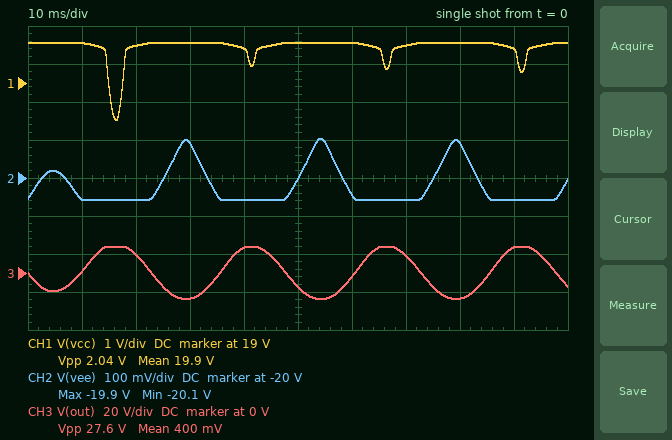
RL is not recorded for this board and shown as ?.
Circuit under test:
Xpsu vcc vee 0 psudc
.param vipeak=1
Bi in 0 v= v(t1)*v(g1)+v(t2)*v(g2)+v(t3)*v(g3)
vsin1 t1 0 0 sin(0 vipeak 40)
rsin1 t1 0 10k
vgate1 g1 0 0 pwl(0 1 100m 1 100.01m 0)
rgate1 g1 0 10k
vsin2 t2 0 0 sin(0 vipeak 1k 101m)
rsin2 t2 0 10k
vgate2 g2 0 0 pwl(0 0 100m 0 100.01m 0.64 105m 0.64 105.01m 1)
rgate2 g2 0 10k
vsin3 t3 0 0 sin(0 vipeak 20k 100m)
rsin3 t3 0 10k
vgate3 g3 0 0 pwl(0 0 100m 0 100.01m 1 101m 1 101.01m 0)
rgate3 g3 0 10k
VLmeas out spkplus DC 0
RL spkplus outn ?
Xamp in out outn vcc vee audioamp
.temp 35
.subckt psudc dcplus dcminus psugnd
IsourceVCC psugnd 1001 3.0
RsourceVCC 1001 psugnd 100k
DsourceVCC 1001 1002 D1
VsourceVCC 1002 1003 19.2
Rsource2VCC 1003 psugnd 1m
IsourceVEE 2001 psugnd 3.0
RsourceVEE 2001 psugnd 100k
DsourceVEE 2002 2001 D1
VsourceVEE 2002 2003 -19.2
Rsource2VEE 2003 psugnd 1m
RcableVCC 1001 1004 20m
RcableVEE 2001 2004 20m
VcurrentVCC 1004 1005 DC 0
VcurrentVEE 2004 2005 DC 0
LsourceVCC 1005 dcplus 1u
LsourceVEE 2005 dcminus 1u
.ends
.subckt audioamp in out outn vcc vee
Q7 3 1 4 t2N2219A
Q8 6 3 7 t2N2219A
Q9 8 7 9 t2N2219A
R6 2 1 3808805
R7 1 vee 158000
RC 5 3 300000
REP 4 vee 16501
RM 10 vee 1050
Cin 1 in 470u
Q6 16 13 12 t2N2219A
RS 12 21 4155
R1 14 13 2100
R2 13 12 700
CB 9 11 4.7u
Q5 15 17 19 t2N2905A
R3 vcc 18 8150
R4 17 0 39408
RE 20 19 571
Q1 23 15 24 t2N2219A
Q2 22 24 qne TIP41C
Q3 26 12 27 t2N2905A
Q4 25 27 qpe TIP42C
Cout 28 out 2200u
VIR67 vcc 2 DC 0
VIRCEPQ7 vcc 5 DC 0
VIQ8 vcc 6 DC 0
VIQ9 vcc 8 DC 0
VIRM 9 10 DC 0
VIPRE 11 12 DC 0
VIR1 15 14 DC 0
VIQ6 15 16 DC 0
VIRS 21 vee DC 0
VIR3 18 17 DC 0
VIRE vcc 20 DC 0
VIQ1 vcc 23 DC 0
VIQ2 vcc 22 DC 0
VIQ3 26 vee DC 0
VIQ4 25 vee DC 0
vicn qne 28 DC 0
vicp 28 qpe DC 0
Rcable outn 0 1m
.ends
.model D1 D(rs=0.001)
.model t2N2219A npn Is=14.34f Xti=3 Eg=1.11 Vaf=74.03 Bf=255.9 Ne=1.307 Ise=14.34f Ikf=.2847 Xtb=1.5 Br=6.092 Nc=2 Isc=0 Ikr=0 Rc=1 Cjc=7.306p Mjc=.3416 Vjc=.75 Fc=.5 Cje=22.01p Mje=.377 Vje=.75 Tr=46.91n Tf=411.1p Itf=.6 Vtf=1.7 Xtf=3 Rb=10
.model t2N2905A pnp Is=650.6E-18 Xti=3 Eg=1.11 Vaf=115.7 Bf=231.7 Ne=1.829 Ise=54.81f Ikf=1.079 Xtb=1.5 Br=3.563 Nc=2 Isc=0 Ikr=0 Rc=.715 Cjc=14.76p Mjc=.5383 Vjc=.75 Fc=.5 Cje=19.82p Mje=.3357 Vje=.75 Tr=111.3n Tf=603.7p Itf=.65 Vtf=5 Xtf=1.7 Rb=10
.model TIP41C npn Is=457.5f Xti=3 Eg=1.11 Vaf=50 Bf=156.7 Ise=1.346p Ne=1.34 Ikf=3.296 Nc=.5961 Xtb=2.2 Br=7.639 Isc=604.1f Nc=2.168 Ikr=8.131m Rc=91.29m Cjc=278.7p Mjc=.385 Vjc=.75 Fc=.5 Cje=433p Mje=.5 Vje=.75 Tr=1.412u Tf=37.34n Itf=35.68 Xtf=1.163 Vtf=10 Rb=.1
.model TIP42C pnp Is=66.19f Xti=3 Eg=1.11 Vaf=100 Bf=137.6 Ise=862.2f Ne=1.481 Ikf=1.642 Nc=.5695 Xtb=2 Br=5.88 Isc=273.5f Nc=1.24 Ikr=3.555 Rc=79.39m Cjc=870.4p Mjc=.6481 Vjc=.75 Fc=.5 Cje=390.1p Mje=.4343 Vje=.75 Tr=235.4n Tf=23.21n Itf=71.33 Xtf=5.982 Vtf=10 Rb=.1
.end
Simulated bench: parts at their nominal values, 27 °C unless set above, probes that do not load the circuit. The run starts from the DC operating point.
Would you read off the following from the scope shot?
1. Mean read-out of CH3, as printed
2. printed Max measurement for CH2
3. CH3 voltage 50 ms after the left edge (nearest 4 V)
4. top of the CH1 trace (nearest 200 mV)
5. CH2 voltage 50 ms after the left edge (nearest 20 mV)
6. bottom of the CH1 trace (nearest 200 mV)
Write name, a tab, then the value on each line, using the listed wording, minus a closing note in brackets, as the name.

Mean read-out of CH3, as printed	400 mV
printed Max measurement for CH2	-19.9 V
CH3 voltage 50 ms after the left edge	-8 V
top of the CH1 trace	20.0 V
CH2 voltage 50 ms after the left edge	-20.00 V
bottom of the CH1 trace	18.0 V
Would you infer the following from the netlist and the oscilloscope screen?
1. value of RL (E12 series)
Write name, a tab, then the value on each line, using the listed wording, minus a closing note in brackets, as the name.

value of RL	4.7 Ω
